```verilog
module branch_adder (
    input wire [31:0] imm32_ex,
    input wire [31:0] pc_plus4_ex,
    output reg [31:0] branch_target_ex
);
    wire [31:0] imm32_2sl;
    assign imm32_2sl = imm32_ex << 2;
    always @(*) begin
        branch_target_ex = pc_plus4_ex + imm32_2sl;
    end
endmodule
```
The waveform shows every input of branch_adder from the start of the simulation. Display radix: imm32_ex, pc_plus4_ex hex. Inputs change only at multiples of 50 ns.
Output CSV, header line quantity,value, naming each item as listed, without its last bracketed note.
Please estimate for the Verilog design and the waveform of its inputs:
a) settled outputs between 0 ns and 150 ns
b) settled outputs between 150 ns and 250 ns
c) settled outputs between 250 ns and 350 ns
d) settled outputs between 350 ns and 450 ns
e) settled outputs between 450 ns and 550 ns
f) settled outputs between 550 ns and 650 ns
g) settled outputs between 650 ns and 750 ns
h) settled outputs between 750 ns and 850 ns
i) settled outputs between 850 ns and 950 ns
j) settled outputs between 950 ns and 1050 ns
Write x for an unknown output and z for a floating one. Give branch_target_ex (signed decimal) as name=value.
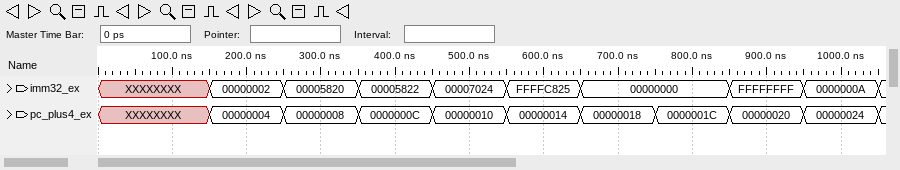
quantity,value
settled outputs between 0 ns and 150 ns,branch_target_ex=x
settled outputs between 150 ns and 250 ns,branch_target_ex=12
settled outputs between 250 ns and 350 ns,branch_target_ex=90248
settled outputs between 350 ns and 450 ns,branch_target_ex=90260
settled outputs between 450 ns and 550 ns,branch_target_ex=114848
settled outputs between 550 ns and 650 ns,branch_target_ex=-57176
settled outputs between 650 ns and 750 ns,branch_target_ex=24
settled outputs between 750 ns and 850 ns,branch_target_ex=28
settled outputs between 850 ns and 950 ns,branch_target_ex=28
settled outputs between 950 ns and 1050 ns,branch_target_ex=76
